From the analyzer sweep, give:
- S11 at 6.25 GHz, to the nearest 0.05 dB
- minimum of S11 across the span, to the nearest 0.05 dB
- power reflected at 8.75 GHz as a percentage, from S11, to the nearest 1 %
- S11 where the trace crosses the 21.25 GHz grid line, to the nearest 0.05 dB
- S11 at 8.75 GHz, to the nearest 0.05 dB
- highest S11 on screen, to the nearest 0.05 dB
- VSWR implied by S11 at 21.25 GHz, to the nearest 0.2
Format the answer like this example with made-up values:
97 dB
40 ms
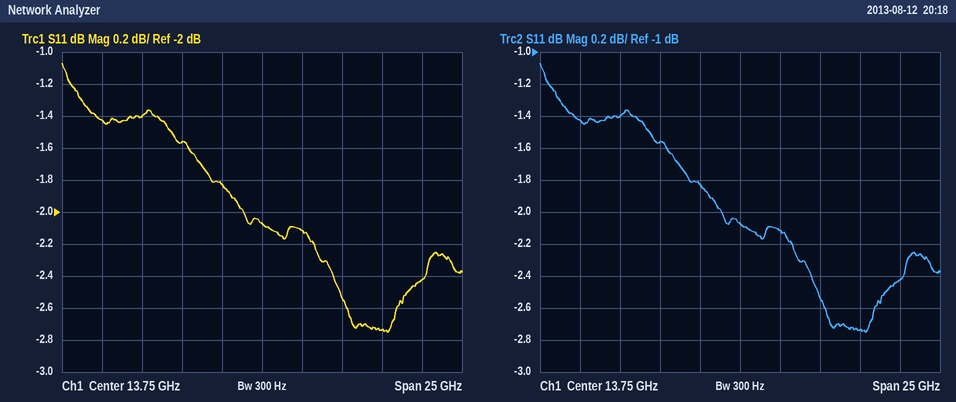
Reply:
-1.40 dB
-2.75 dB
70 %
-2.75 dB
-1.55 dB
-1.05 dB
6.4
